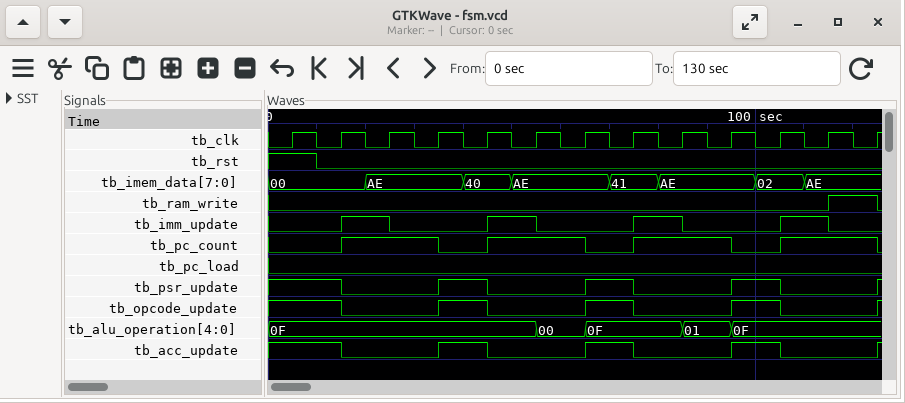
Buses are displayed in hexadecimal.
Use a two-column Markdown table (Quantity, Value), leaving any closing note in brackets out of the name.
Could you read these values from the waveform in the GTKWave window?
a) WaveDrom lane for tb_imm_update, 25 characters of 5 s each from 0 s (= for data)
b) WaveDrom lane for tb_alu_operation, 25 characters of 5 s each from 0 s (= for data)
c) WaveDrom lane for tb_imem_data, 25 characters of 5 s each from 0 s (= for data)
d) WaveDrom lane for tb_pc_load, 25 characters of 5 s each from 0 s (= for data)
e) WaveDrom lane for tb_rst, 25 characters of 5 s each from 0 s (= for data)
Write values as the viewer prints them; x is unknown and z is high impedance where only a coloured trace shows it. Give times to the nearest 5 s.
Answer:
| Quantity | Value |
|---|---|
| WaveDrom lane for tb_imm_update, 25 characters of 5 s each from 0 s | {name: 'tb_imm_update', wave: '0..1.0...1.0...1.0...1.0.'} |
| WaveDrom lane for tb_alu_operation, 25 characters of 5 s each from 0 s | {name: 'tb_alu_operation', wave: '=..........=.=...=.=.....', data: '0F 00 0F 01 0F'} |
| WaveDrom lane for tb_imem_data, 25 characters of 5 s each from 0 s | {name: 'tb_imem_data', wave: '=...=...=.=...=.=...=.=..', data: '00 AE 40 AE 41 AE 02 AE'} |
| WaveDrom lane for tb_pc_load, 25 characters of 5 s each from 0 s | {name: 'tb_pc_load', wave: '0........................'} |
| WaveDrom lane for tb_rst, 25 characters of 5 s each from 0 s | {name: 'tb_rst', wave: '1.0......................'} |
